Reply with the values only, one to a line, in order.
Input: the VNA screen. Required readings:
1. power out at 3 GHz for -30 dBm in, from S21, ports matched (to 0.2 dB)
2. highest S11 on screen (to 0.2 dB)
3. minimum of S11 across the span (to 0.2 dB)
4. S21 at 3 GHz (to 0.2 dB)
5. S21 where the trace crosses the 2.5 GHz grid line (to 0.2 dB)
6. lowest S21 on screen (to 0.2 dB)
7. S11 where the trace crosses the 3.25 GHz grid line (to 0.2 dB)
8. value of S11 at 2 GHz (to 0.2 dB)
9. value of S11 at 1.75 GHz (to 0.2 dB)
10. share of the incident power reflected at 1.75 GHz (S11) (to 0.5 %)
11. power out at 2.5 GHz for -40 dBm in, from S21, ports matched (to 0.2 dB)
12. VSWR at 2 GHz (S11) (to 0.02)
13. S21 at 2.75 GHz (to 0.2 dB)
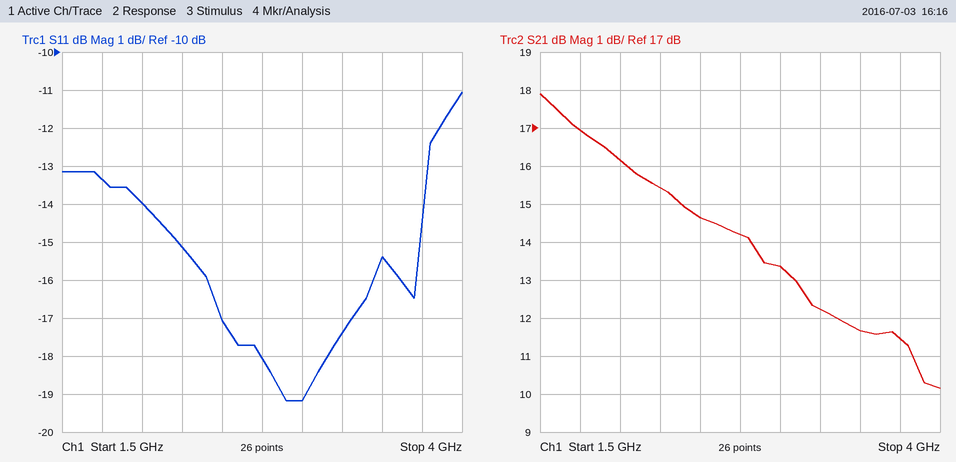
-16.6 dBm
-11.0 dB
-19.2 dB
13.4 dB
14.6 dB
10.2 dB
-17.4 dB
-14.0 dB
-13.4 dB
4.5 %
-25.4 dBm
1.50
14.2 dB
